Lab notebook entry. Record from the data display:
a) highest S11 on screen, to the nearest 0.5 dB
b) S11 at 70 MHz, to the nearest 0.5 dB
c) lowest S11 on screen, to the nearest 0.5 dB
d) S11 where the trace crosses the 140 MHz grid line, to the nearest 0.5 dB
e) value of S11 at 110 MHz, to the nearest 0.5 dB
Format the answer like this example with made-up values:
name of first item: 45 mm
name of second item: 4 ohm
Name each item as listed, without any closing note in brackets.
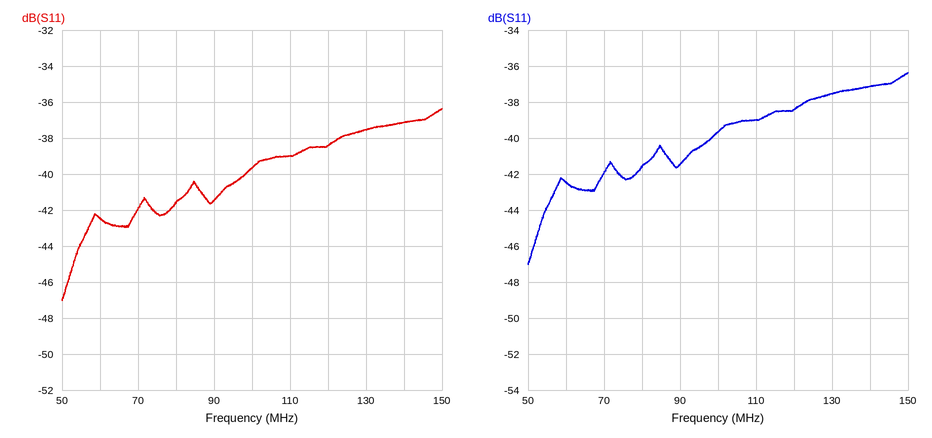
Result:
highest S11 on screen, to the nearest 0.5 dB: -36.5 dB
S11 at 70 MHz, to the nearest 0.5 dB: -42.0 dB
lowest S11 on screen, to the nearest 0.5 dB: -47.0 dB
S11 where the trace crosses the 140 MHz grid line, to the nearest 0.5 dB: -37.0 dB
value of S11 at 110 MHz, to the nearest 0.5 dB: -39.0 dB
